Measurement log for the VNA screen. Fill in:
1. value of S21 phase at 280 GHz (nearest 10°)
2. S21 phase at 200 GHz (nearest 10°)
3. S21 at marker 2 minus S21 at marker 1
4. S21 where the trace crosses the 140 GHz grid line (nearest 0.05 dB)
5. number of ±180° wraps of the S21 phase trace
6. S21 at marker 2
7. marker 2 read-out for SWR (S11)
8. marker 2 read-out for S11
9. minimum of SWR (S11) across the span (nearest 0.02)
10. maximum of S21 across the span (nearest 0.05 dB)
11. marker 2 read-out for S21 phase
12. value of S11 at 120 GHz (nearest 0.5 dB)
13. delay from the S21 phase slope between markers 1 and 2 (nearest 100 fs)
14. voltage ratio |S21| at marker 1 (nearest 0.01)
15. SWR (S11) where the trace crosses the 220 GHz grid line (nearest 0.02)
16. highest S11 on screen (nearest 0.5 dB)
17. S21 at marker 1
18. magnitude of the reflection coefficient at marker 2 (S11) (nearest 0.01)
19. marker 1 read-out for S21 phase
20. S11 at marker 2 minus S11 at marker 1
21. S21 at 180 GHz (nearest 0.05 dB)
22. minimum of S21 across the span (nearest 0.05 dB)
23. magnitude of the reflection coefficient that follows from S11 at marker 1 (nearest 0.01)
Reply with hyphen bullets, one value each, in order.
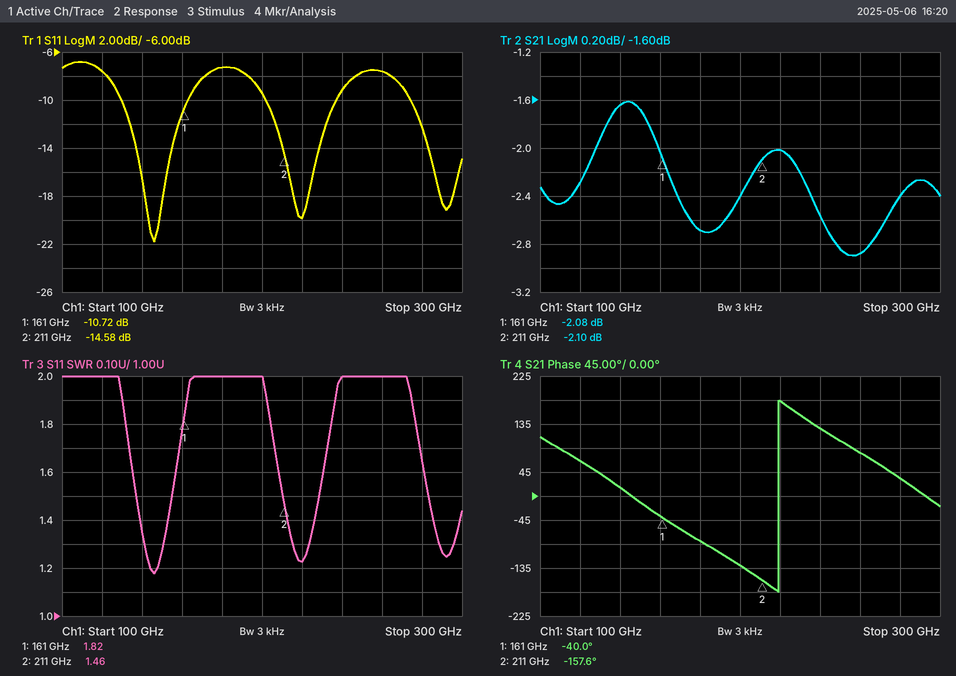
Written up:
- 30°
- -130°
- -0.02 dB
- -1.65 dB
- 1
- -2.10 dB
- 1.46
- -14.58 dB
- 1.18
- -1.60 dB
- -157.6°
- -7.5 dB
- 6.5 ps
- 0.79
- 1.22
- -7.0 dB
- -2.08 dB
- 0.19
- -40.0°
- -3.86 dB
- -2.70 dB
- -2.90 dB
- 0.29
